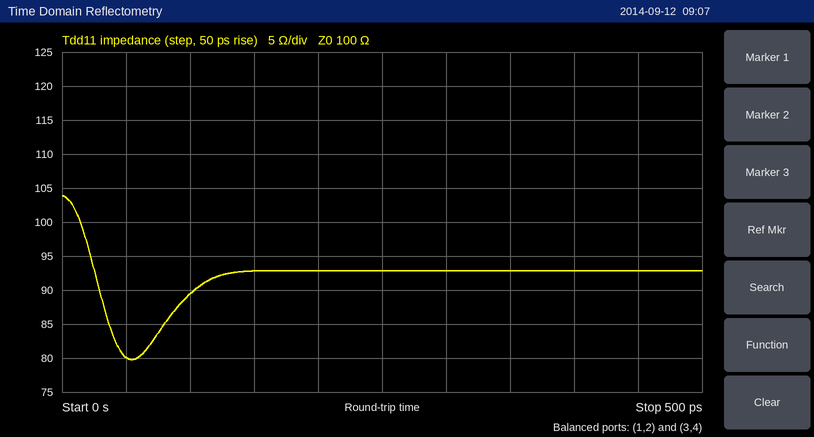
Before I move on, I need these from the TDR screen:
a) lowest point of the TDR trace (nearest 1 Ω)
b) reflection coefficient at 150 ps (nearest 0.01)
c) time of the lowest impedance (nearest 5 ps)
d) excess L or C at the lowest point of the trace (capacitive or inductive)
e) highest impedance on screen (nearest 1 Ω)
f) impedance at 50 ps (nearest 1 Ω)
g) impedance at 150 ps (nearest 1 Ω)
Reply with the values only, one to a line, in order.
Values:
80 Ω
-0.04
55 ps
capacitive
104 Ω
80 Ω
93 Ω
